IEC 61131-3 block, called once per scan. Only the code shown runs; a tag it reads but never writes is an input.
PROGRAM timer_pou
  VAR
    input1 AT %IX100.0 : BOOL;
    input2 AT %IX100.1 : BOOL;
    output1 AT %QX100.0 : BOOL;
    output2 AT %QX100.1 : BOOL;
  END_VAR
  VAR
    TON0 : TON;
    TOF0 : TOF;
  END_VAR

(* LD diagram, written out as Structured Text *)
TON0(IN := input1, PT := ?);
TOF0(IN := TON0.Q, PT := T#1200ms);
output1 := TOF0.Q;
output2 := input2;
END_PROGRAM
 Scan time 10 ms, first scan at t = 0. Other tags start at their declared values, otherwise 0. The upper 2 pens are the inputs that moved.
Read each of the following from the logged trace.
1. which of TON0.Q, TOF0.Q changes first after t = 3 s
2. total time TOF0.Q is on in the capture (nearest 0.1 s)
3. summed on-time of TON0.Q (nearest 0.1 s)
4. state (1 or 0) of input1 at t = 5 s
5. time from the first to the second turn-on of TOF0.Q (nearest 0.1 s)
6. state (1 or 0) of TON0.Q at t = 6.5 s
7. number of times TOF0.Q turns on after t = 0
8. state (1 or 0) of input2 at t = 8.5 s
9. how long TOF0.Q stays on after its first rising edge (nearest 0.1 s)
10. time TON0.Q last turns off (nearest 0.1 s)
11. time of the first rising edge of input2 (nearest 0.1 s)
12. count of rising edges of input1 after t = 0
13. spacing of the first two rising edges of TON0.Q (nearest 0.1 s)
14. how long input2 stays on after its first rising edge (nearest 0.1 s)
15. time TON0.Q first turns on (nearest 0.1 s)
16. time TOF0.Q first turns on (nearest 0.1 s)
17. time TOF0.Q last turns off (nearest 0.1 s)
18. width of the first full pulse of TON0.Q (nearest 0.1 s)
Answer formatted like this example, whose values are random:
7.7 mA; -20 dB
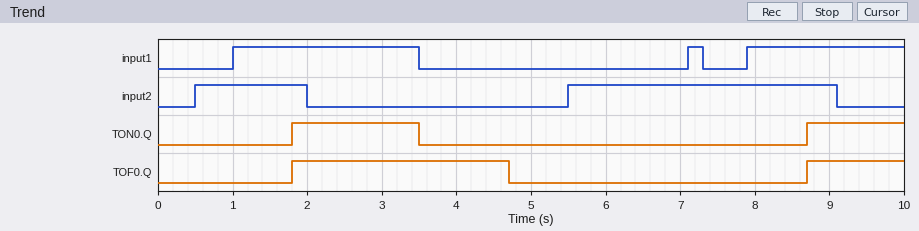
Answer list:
TON0.Q; 4.2 s; 3.0 s; 0; 6.9 s; 0; 2; 1; 2.9 s; 3.5 s; 0.5 s; 3; 6.9 s; 1.5 s; 1.8 s; 1.8 s; 4.7 s; 1.7 s
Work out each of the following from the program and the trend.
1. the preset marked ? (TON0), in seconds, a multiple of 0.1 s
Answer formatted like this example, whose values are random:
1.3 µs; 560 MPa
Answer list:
0.8 s
